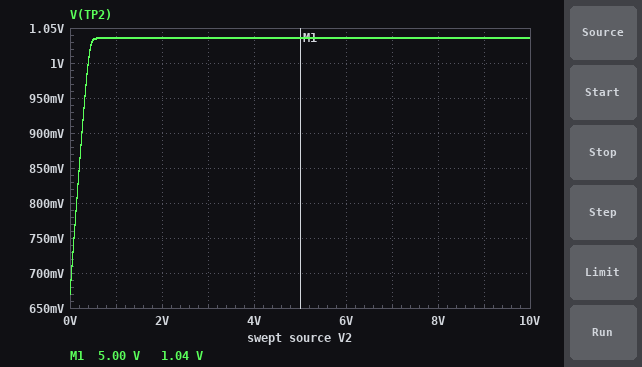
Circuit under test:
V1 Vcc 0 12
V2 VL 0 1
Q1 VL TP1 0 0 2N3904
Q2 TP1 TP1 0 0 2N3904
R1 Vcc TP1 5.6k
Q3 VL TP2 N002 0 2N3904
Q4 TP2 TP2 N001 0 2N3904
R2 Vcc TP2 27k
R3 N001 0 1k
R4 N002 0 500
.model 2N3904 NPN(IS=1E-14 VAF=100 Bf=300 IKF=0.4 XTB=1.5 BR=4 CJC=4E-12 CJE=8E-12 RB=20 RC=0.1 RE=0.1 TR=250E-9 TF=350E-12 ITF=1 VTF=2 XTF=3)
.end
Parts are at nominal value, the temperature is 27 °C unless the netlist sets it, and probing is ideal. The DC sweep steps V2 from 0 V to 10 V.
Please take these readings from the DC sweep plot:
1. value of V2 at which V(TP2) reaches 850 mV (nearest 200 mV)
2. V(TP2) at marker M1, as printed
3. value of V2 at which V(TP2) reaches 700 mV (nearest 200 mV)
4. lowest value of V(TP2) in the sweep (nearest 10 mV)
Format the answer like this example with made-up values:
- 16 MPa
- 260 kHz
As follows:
- 200 mV
- 1.04 V
- 0 V
- 670 mV
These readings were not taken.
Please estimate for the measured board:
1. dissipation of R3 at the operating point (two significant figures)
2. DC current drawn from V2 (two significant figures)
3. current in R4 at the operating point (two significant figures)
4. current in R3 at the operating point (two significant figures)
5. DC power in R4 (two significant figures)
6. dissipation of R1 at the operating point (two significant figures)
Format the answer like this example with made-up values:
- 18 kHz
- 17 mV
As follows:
- 160 µW
- 2.8 mA
- 770 µA
- 400 µA
- 300 µW
- 23 mW
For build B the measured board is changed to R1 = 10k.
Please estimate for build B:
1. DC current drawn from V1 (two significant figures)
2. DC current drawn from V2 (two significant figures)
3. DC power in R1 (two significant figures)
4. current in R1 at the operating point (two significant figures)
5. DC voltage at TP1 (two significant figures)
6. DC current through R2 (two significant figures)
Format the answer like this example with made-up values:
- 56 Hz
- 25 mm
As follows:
- 1.5 mA
- 1.9 mA
- 13 mW
- 1.1 mA
- 660 mV
- 410 µA
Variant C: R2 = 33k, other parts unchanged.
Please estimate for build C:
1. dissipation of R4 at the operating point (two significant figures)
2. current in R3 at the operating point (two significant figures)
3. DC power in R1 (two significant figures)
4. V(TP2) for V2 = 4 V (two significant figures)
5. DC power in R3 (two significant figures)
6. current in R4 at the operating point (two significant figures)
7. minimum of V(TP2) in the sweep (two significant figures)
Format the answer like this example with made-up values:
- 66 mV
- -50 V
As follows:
- 200 µW
- 330 µA
- 23 mW
- 960 mV
- 110 µW
- 630 µA
- 660 mV
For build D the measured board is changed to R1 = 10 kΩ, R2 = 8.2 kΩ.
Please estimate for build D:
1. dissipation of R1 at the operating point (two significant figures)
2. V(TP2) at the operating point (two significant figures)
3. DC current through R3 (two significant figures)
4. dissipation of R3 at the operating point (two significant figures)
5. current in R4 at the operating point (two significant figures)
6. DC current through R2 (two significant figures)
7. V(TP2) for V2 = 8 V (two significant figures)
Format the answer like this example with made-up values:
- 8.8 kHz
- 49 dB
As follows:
- 13 mW
- 1.7 V
- 1.0 mA
- 1.0 mW
- 1.9 mA
- 1.3 mA
- 1.9 V
